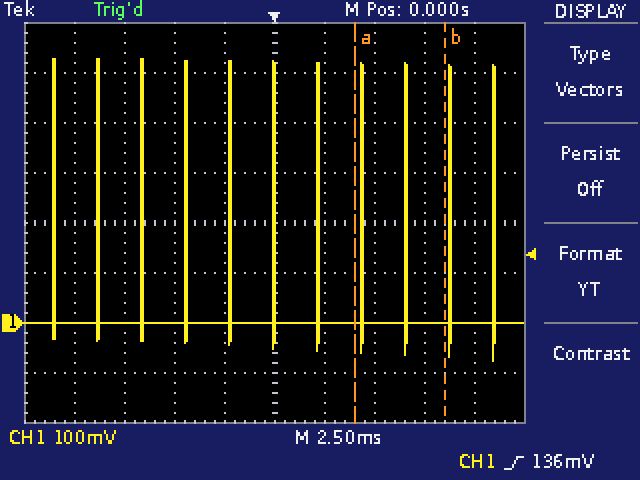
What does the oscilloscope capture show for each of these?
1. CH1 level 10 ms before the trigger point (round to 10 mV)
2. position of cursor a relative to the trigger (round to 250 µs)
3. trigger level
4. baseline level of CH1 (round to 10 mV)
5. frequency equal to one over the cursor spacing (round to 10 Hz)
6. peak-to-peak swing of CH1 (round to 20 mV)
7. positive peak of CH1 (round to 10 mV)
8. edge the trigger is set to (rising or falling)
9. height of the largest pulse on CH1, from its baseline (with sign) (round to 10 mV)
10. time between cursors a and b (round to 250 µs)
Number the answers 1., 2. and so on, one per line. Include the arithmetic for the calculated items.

1. 0 mV
2. +4.00 ms
3. 136 mV
4. 0 mV
5. 1 / 4.50 ms ≈ 220 Hz
6. 600 mV
7. 530 mV
8. rising
9. 530 mV − (0 mV) = +530 mV
10. 4.50 ms
